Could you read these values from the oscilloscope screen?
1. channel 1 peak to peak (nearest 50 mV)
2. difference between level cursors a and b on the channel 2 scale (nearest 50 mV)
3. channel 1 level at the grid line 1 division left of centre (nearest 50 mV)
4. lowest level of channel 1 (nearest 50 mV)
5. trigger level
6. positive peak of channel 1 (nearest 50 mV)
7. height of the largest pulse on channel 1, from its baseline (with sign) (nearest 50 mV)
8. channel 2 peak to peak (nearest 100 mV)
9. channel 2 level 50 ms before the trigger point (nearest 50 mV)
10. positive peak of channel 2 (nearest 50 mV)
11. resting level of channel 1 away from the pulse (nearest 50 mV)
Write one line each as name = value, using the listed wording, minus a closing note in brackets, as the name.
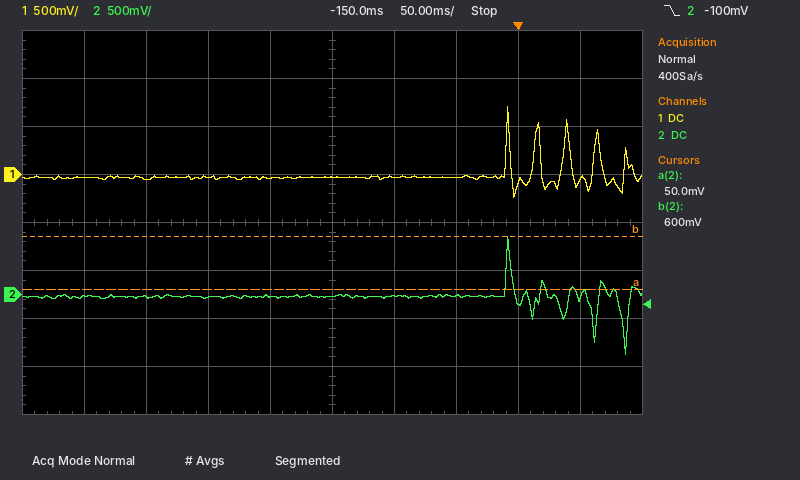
channel 1 peak to peak = 950 mV
difference between level cursors a and b on the channel 2 scale = 550 mV
channel 1 level at the grid line 1 division left of centre = -50 mV
lowest level of channel 1 = -250 mV
trigger level = -100 mV
positive peak of channel 1 = 700 mV
height of the largest pulse on channel 1, from its baseline (with sign) = +750 mV
channel 2 peak to peak = 1.20 V
channel 2 level 50 ms before the trigger point = 0 mV
positive peak of channel 2 = 600 mV
resting level of channel 1 away from the pulse = -50 mV
